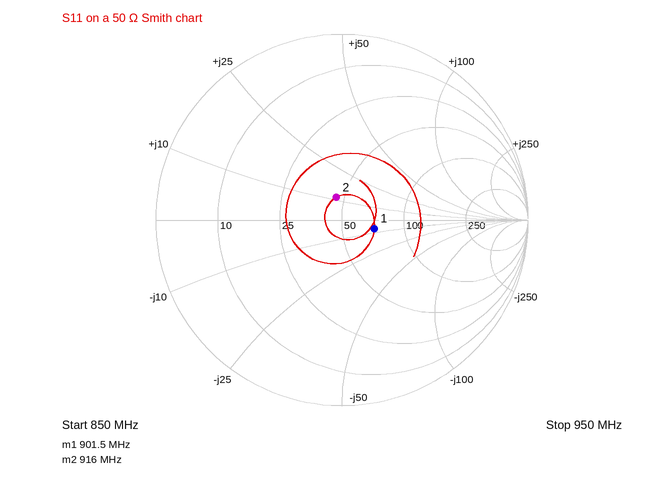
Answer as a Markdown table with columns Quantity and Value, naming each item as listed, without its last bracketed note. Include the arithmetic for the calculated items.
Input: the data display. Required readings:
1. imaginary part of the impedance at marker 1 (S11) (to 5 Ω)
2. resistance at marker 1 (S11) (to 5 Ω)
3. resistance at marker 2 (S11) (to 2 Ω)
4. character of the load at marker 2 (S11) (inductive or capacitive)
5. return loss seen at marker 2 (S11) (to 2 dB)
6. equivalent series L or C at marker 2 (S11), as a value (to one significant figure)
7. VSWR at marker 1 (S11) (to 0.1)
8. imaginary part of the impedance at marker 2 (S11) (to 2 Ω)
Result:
| Quantity | Value |
|---|---|
| imaginary part of the impedance at marker 1 (S11) | -5 Ω |
| resistance at marker 1 (S11) | 70 Ω |
| resistance at marker 2 (S11) | 46 Ω |
| character of the load at marker 2 (S11) | inductive |
| return loss seen at marker 2 (S11) | 18 dB |
| equivalent series L or C at marker 2 (S11), as a value | L = 12 Ω/(2π × 916 MHz) ≈ 2 nH |
| VSWR at marker 1 (S11) | 1.4 |
| imaginary part of the impedance at marker 2 (S11) | +12 Ω |
